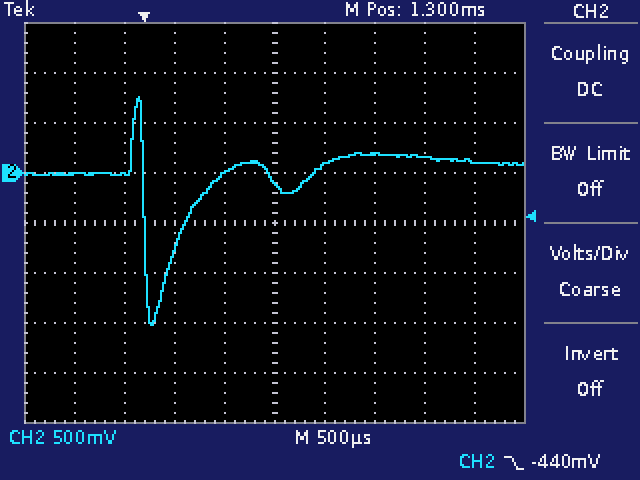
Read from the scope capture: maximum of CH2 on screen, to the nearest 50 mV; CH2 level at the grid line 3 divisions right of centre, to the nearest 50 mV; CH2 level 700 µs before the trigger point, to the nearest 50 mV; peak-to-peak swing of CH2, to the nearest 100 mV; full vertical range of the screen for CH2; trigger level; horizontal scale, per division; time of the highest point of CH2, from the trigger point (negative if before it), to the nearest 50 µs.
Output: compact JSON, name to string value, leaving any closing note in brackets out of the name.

{"maximum of CH2 on screen, to the nearest 50 mV": "750 mV", "CH2 level at the grid line 3 divisions right of centre, to the nearest 50 mV": "150 mV", "CH2 level 700 µs before the trigger point, to the nearest 50 mV": "0 mV", "peak-to-peak swing of CH2, to the nearest 100 mV": "2.30 V", "full vertical range of the screen for CH2": "4 V", "trigger level": "-440 mV", "horizontal scale, per division": "500 µs", "time of the highest point of CH2, from the trigger point (negative if before it), to the nearest 50 µs": "-50 µs"}
